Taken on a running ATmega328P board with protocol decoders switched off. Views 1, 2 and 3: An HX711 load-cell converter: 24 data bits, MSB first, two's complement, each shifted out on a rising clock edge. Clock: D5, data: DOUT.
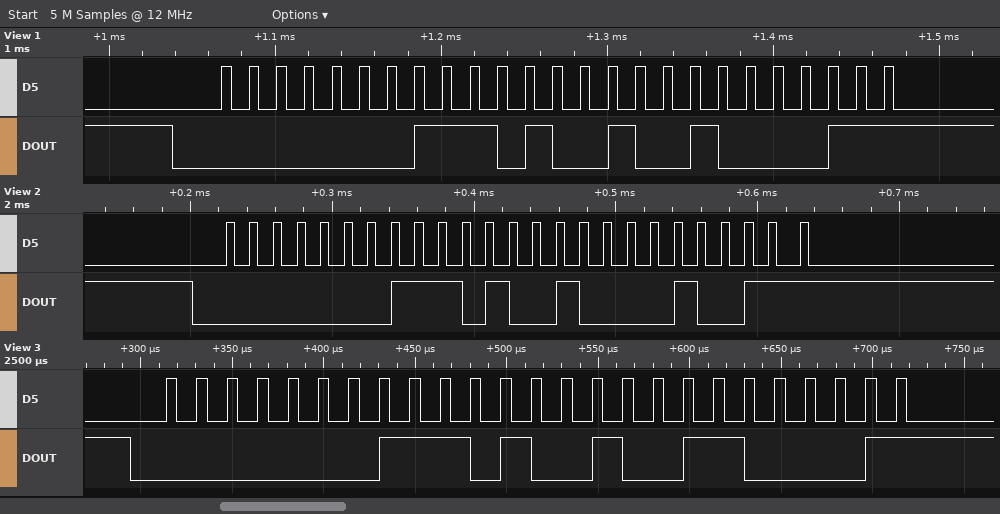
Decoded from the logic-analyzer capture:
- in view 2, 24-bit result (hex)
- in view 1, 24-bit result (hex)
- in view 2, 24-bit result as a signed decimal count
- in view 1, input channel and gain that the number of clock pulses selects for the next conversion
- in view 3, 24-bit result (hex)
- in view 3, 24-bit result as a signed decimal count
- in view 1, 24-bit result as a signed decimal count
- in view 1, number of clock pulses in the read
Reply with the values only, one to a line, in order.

0x01D213
0x01D243
119315
channel A, gain 128
0x01D261
119393
119363
25
